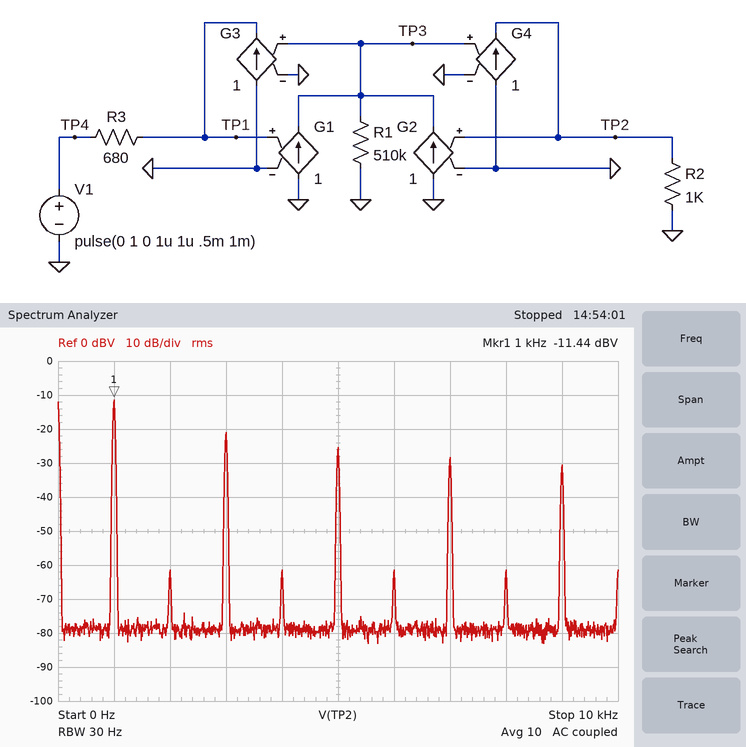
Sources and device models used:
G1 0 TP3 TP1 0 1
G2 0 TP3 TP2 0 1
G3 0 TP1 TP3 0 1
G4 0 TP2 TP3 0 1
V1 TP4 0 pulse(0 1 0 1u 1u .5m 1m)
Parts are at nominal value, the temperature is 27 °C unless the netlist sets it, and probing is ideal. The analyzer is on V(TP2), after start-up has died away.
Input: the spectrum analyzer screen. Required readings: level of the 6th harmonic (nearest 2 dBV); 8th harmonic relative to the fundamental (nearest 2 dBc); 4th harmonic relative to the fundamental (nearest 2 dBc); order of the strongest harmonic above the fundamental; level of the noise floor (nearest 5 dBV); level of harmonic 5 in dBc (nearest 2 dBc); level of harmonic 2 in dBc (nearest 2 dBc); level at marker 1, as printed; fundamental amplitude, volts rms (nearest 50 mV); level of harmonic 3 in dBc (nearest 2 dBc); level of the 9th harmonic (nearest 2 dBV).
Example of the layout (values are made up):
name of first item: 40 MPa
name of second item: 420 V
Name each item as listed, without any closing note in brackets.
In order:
level of the 6th harmonic: -62 dBV
8th harmonic relative to the fundamental: -50 dBc
4th harmonic relative to the fundamental: -50 dBc
order of the strongest harmonic above the fundamental: 3
level of the noise floor: -80 dBV
level of harmonic 5 in dBc: -14 dBc
level of harmonic 2 in dBc: -50 dBc
level at marker 1, as printed: -11.44 dBV
fundamental amplitude, volts rms: 250 mV
level of harmonic 3 in dBc: -10 dBc
level of the 9th harmonic: -30 dBV
